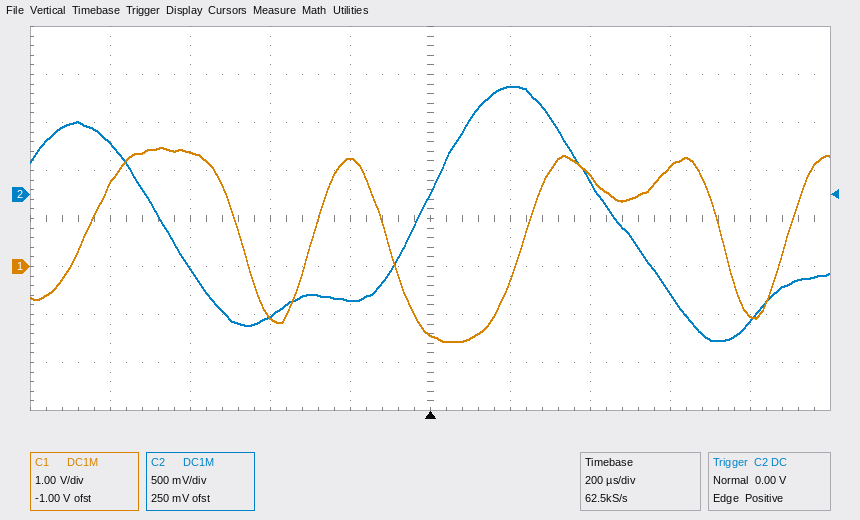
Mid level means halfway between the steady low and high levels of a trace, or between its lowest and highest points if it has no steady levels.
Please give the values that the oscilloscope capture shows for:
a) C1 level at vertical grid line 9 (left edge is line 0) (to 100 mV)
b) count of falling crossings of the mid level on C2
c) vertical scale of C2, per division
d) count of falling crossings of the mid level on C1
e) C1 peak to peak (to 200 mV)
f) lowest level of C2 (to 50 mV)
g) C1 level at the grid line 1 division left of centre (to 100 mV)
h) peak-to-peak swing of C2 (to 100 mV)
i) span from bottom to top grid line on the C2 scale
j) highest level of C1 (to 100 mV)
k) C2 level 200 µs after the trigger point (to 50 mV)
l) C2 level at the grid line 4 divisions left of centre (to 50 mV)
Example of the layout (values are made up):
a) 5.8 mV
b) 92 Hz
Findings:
a) -1.0 V
b) 2
c) 500 mV
d) 3
e) 4.0 V
f) -1.50 V
g) 2.2 V
h) 2.60 V
i) 4 V
j) 2.5 V
k) 1.10 V
l) 550 mV
